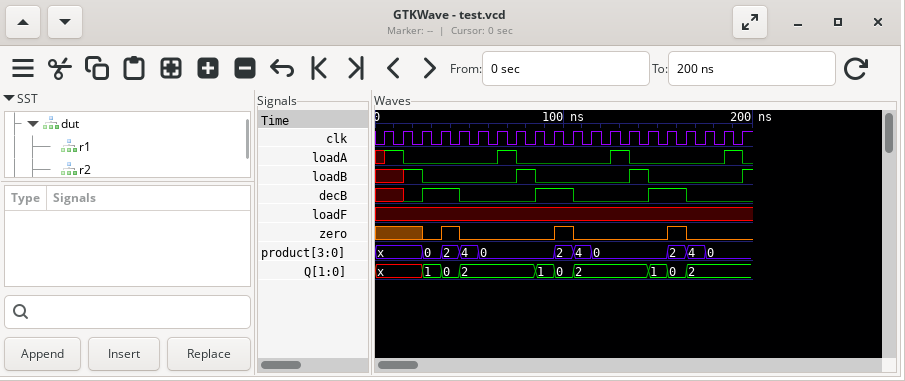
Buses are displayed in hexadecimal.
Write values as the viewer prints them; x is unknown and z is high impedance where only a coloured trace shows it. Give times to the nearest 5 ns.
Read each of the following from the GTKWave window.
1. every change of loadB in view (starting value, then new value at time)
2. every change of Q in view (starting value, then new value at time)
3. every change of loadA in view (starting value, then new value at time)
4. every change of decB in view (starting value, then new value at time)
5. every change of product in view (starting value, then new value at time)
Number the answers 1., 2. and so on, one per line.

1. x, 1 at 15 ns, 0 at 25 ns, 1 at 75 ns, 0 at 85 ns, 1 at 135 ns, 0 at 145 ns, 1 at 195 ns
2. x, 1 at 25 ns, 0 at 35 ns, 2 at 45 ns, 1 at 85 ns, 0 at 95 ns, 2 at 105 ns, 1 at 145 ns, 0 at 155 ns, 2 at 165 ns
3. x, 1 at 5 ns, 0 at 15 ns, 1 at 65 ns, 0 at 75 ns, 1 at 125 ns, 0 at 135 ns, 1 at 185 ns, 0 at 195 ns
4. x, 0 at 15 ns, 1 at 25 ns, 0 at 45 ns, 1 at 85 ns, 0 at 105 ns, 1 at 145 ns, 0 at 165 ns
5. x, 0 at 25 ns, 2 at 35 ns, 4 at 45 ns, 0 at 55 ns, 2 at 95 ns, 4 at 105 ns, 0 at 115 ns, 2 at 155 ns, 4 at 165 ns, 0 at 175 ns
